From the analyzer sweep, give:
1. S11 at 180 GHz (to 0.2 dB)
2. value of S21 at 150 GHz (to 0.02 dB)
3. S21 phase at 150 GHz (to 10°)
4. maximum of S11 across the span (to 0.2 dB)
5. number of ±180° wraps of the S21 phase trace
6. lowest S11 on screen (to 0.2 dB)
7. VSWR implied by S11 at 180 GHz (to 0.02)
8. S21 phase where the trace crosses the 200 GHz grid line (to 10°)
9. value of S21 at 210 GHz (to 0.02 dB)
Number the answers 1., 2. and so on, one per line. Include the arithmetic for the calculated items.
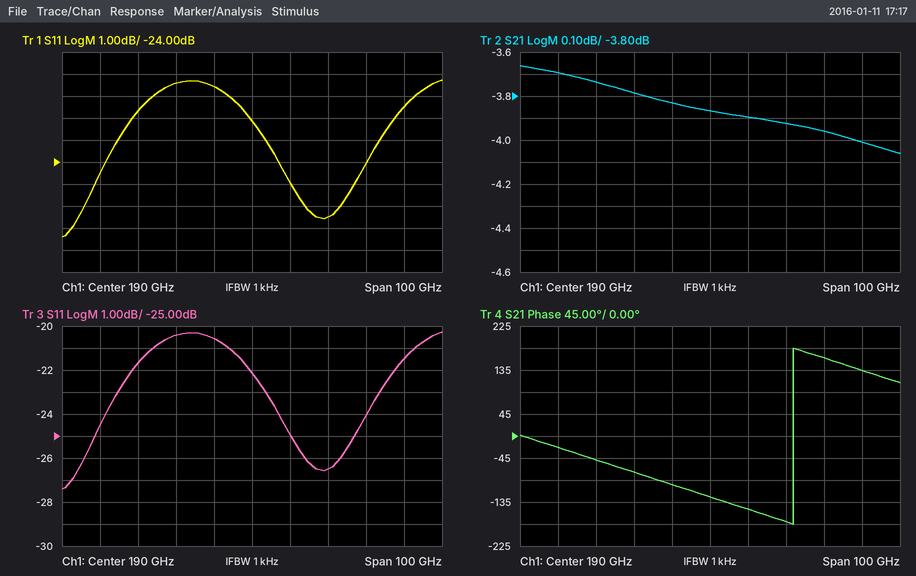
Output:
1. -20.6 dB
2. -3.70 dB
3. -20°
4. -20.2 dB
5. 1
6. -27.4 dB
7. |Γ| = 10^(-20.6/20) = 0.0933; VSWR = (1 + 0.0933)/(1 − 0.0933) ≈ 1.21, so 1.20 to the nearest 0.02
8. -150°
9. -3.92 dB
